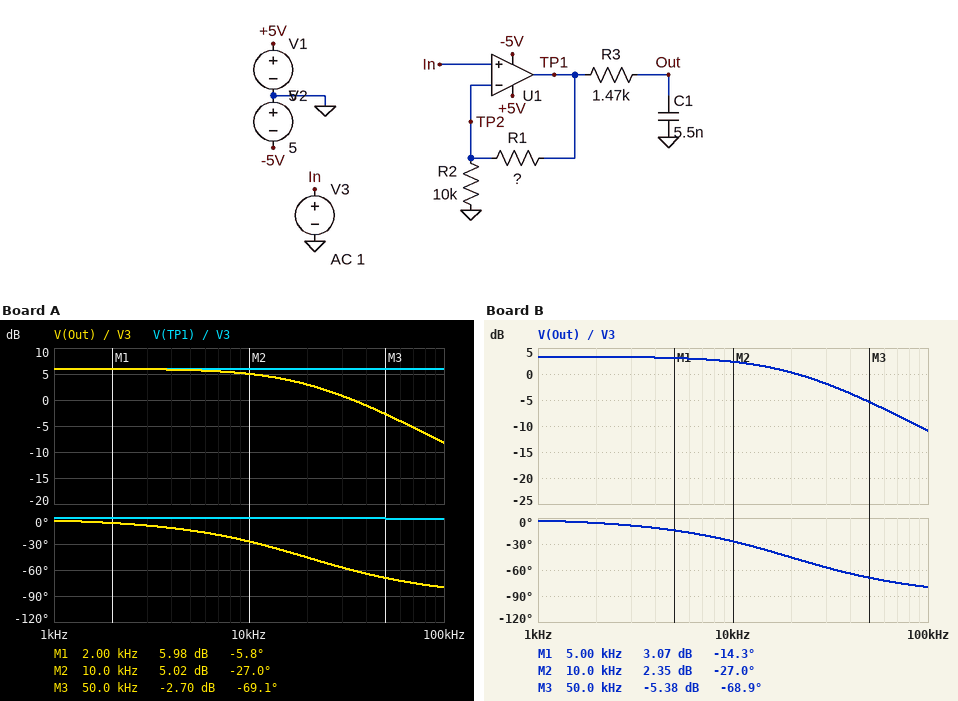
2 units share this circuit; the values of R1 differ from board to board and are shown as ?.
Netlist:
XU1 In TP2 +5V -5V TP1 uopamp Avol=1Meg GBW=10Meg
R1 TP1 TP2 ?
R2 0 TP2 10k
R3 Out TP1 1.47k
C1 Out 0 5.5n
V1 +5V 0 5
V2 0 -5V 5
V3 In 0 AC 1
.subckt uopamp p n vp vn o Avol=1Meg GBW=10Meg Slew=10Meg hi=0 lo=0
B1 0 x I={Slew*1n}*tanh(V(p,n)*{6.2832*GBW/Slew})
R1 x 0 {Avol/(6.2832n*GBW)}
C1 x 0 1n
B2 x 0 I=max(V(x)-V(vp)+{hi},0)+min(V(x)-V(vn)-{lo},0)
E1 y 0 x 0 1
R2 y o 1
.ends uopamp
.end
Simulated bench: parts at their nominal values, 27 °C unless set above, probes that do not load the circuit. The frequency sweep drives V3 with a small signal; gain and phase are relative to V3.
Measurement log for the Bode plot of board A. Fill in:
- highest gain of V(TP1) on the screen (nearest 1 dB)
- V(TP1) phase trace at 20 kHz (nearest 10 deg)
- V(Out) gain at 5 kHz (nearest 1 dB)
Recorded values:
6 dB
0 deg
6 dB
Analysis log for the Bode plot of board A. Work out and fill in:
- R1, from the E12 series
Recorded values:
10 kΩ
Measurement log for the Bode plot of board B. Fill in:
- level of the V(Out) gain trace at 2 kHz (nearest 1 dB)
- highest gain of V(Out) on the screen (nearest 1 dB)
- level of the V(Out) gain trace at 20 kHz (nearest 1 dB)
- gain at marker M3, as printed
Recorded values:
3 dB
3 dB
0 dB
-5.38 dB
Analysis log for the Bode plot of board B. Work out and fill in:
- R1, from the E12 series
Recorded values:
4.7 kΩ
